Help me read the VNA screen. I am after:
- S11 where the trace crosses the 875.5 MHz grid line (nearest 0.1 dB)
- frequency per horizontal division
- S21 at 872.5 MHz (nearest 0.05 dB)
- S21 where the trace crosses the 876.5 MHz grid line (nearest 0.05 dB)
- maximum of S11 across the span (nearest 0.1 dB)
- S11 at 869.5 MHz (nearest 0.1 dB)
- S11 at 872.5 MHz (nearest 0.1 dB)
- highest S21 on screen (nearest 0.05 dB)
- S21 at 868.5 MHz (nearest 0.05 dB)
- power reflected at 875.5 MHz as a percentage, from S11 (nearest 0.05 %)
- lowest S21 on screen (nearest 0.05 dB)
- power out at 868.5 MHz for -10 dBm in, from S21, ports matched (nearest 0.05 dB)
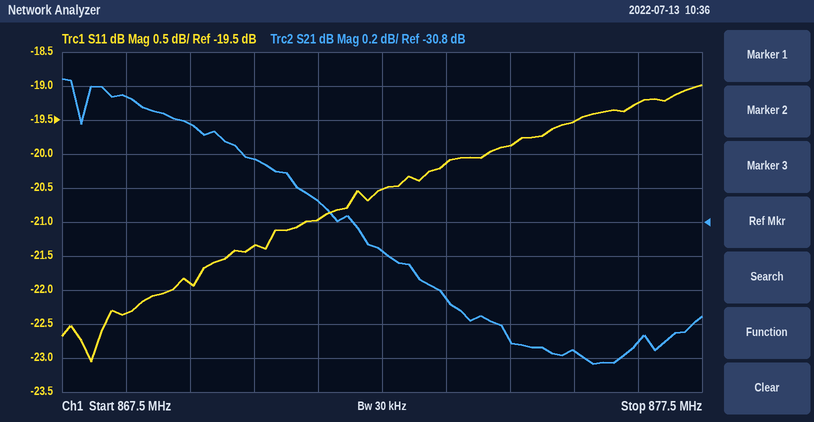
-19.5 dB
1 MHz
-30.95 dB
-31.50 dB
-19.0 dB
-21.9 dB
-20.5 dB
-29.95 dB
-30.05 dB
1.10 %
-31.65 dB
-40.05 dBm
